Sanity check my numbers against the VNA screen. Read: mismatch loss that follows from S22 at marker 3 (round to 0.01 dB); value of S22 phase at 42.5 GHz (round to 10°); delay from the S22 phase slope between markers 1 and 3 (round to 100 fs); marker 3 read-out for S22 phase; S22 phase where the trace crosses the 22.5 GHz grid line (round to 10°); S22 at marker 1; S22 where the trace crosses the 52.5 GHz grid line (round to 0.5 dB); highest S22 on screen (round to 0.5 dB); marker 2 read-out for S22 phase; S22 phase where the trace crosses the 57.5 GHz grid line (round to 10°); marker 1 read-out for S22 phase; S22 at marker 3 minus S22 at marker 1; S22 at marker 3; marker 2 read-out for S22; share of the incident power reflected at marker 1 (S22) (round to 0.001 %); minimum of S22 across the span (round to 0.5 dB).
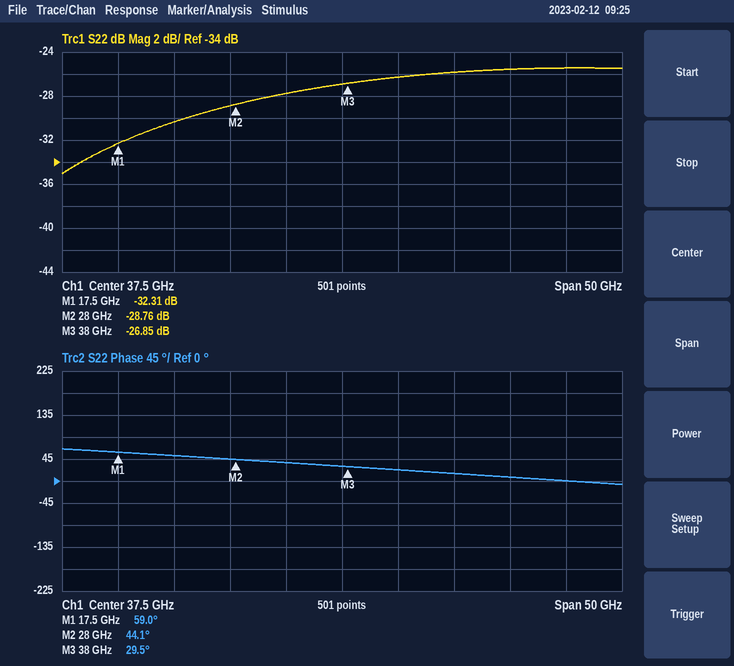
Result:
0.01 dB
20°
4.0 ps
29.5°
50°
-32.31 dB
-25.5 dB
-25.5 dB
44.1°
0°
59.0°
5.46 dB
-26.85 dB
-28.76 dB
0.059 %
-35.0 dB
